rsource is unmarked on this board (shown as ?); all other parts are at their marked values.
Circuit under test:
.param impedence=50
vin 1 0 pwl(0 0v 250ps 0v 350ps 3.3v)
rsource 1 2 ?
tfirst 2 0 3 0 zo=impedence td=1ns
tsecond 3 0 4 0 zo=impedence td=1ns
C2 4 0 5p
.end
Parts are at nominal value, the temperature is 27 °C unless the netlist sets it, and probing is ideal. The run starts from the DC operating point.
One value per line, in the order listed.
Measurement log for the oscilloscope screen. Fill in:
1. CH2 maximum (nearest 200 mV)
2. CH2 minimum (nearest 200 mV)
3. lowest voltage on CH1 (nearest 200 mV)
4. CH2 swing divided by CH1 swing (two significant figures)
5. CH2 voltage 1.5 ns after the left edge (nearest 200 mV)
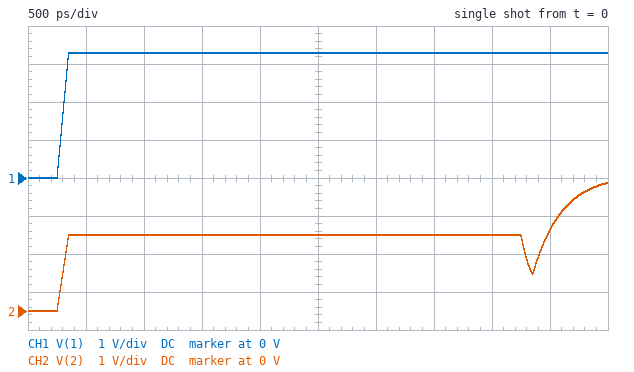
3.4 V
0 V
0 V
1.0
2.0 V
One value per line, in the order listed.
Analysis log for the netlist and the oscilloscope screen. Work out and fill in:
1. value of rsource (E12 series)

33 Ω
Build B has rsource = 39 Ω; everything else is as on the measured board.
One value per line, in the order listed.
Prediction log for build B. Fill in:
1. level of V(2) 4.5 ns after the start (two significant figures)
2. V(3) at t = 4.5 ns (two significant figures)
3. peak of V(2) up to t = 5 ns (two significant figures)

2.0 V
3.7 V
3.3 V
